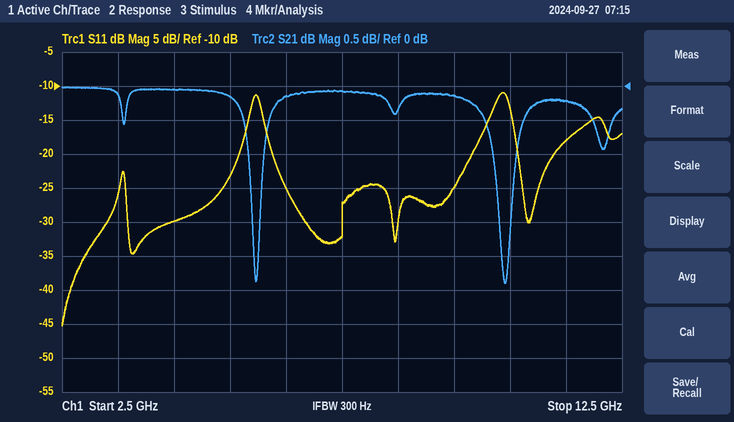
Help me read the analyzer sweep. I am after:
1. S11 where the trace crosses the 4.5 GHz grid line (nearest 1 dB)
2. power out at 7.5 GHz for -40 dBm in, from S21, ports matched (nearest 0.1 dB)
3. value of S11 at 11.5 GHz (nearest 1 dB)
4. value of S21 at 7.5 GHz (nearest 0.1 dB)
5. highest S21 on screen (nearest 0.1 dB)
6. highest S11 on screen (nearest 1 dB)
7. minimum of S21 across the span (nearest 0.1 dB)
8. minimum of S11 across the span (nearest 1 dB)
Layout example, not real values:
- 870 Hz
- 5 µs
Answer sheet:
- -30 dB
- -40.1 dBm
- -18 dB
- -0.1 dB
- 0.0 dB
- -11 dB
- -2.9 dB
- -45 dB
